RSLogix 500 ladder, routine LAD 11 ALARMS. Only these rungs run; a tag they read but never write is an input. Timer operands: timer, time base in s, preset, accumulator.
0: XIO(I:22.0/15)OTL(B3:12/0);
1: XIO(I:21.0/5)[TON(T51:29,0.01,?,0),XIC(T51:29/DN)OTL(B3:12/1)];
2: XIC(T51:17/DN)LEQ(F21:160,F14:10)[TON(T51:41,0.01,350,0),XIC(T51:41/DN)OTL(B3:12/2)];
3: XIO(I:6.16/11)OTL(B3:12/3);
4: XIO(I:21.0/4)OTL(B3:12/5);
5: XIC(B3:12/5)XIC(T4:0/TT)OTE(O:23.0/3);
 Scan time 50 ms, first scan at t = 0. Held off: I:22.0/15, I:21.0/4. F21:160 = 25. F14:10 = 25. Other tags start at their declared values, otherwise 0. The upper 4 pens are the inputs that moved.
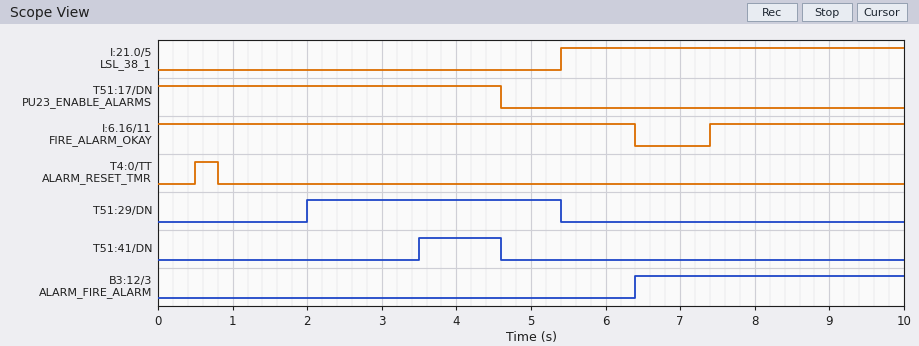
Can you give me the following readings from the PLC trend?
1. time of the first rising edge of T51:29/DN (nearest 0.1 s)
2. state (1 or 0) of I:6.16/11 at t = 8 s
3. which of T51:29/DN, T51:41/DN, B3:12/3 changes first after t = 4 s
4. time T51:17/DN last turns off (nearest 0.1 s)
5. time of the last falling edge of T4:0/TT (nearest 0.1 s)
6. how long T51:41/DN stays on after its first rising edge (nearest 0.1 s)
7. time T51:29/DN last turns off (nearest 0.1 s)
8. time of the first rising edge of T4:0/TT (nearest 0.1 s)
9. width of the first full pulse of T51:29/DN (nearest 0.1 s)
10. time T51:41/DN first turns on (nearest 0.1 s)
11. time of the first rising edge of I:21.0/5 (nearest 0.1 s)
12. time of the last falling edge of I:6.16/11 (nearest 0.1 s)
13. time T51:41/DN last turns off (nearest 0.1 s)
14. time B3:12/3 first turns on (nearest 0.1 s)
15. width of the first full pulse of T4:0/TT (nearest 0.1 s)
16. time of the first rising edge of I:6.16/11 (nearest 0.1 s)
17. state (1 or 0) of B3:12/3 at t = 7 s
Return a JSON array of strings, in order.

["2.0 s", "1", "T51:41/DN", "4.6 s", "0.8 s", "1.1 s", "5.4 s", "0.5 s", "3.4 s", "3.5 s", "5.4 s", "6.4 s", "4.6 s", "6.4 s", "0.3 s", "7.4 s", "1"]
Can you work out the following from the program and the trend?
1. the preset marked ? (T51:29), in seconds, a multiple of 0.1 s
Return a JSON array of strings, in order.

["2.0 s"]
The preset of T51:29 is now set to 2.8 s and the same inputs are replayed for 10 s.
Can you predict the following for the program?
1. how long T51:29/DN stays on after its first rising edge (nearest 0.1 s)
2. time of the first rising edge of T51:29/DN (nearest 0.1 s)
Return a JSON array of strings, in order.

["2.6 s", "2.8 s"]
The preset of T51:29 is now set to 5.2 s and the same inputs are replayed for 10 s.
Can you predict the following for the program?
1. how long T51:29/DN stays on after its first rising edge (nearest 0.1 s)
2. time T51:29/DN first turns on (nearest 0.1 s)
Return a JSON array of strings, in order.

["0.2 s", "5.2 s"]
